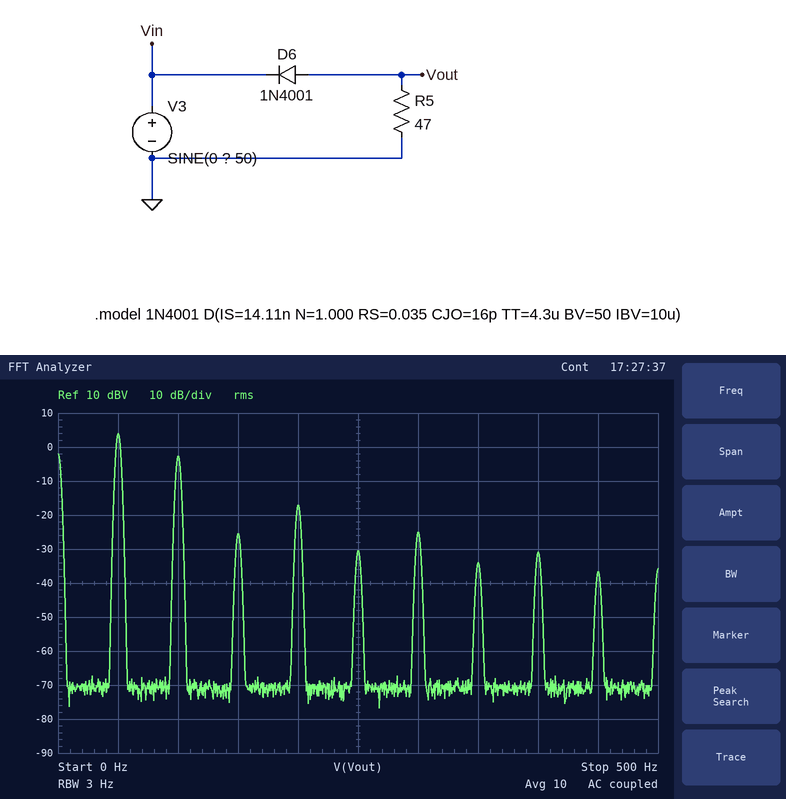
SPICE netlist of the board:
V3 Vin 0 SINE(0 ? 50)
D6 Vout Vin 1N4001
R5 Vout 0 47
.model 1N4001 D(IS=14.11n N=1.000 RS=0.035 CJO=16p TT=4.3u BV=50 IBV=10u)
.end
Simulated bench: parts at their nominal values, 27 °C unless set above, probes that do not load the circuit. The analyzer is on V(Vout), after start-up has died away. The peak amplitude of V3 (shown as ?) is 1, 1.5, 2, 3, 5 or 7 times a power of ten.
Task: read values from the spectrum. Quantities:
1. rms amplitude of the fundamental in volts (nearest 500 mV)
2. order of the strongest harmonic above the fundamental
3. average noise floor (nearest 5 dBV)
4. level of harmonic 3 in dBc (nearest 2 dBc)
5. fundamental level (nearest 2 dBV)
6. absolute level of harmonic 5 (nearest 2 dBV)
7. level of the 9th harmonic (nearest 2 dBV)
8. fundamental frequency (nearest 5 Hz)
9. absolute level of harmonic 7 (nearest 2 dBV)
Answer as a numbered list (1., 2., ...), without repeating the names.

1. 1.5 V
2. 2
3. -70 dBV
4. -30 dBc
5. 4 dBV
6. -30 dBV
7. -36 dBV
8. 50 Hz
9. -34 dBV
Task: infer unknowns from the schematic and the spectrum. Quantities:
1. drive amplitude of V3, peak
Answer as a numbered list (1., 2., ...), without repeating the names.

1. 5 V
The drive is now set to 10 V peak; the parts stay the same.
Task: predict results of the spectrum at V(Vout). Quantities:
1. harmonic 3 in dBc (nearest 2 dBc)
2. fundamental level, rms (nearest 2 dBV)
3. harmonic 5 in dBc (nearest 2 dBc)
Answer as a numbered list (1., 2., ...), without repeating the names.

1. -36 dBc
2. 10 dBV
3. -40 dBc
